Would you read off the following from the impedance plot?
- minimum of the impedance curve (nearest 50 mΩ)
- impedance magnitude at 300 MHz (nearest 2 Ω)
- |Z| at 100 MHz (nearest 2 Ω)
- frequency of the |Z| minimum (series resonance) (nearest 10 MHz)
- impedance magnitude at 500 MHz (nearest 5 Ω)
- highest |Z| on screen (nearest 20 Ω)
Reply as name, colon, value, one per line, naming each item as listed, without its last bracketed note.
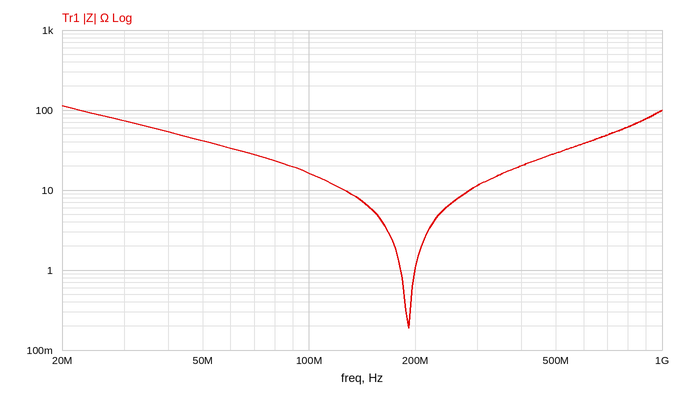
minimum of the impedance curve: 200 mΩ
impedance magnitude at 300 MHz: 12 Ω
|Z| at 100 MHz: 16 Ω
frequency of the |Z| minimum (series resonance): 190 MHz
impedance magnitude at 500 MHz: 30 Ω
highest |Z| on screen: 120 Ω
